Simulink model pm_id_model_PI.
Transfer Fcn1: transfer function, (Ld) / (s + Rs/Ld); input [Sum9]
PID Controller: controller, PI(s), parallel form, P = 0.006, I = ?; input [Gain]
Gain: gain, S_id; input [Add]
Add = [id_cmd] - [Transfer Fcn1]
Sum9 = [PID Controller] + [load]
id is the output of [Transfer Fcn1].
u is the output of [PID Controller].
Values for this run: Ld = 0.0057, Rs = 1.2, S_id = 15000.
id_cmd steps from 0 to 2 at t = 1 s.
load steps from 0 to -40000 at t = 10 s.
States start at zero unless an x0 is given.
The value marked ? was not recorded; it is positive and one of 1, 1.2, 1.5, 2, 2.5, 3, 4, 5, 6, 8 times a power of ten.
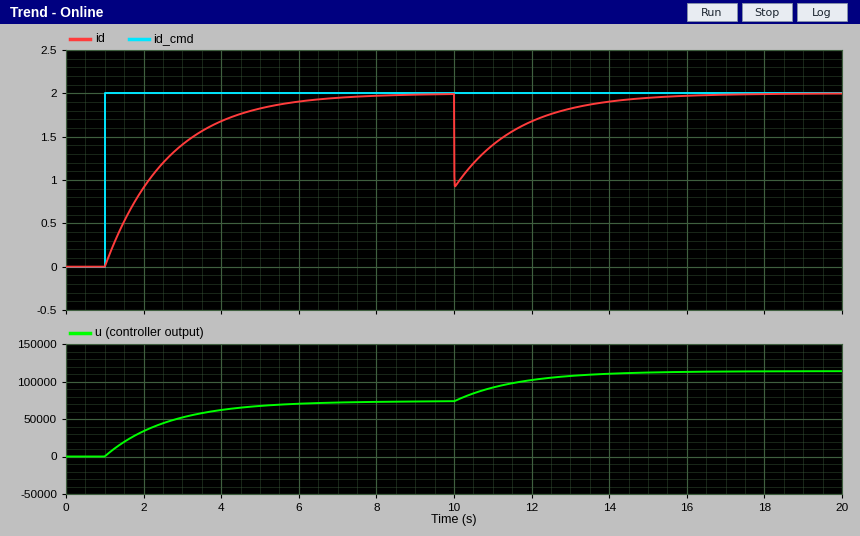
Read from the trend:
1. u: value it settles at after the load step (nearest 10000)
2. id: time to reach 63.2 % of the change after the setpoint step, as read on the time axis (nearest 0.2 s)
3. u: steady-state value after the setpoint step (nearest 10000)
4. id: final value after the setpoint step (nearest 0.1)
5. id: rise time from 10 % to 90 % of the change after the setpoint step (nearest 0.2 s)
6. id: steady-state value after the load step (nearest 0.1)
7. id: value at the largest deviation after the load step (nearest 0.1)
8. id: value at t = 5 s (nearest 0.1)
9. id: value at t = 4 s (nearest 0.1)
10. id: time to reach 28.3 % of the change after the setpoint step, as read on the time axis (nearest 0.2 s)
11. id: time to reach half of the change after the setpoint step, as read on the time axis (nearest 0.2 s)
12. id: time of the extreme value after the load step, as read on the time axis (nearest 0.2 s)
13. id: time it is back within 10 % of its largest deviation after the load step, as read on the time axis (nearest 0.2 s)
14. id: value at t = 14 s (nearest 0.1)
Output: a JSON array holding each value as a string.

["110000", "2.6 s", "70000", "2.0", "3.6 s", "2.0", "0.9", "1.8", "1.7", "1.6 s", "2.2 s", "10.0 s", "13.8 s", "1.9"]
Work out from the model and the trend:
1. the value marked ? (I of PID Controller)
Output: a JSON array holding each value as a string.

["1.5"]
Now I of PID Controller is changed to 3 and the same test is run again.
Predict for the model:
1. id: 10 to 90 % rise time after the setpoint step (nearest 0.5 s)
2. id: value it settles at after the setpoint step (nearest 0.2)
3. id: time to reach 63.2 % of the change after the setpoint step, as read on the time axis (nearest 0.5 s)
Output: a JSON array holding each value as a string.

["2.0 s", "2.0", "2.0 s"]
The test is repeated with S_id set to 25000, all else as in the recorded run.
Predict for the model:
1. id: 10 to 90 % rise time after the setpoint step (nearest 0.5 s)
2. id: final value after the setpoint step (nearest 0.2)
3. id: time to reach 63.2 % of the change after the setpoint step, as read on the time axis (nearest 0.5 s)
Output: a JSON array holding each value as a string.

["2.0 s", "2.0", "2.0 s"]
